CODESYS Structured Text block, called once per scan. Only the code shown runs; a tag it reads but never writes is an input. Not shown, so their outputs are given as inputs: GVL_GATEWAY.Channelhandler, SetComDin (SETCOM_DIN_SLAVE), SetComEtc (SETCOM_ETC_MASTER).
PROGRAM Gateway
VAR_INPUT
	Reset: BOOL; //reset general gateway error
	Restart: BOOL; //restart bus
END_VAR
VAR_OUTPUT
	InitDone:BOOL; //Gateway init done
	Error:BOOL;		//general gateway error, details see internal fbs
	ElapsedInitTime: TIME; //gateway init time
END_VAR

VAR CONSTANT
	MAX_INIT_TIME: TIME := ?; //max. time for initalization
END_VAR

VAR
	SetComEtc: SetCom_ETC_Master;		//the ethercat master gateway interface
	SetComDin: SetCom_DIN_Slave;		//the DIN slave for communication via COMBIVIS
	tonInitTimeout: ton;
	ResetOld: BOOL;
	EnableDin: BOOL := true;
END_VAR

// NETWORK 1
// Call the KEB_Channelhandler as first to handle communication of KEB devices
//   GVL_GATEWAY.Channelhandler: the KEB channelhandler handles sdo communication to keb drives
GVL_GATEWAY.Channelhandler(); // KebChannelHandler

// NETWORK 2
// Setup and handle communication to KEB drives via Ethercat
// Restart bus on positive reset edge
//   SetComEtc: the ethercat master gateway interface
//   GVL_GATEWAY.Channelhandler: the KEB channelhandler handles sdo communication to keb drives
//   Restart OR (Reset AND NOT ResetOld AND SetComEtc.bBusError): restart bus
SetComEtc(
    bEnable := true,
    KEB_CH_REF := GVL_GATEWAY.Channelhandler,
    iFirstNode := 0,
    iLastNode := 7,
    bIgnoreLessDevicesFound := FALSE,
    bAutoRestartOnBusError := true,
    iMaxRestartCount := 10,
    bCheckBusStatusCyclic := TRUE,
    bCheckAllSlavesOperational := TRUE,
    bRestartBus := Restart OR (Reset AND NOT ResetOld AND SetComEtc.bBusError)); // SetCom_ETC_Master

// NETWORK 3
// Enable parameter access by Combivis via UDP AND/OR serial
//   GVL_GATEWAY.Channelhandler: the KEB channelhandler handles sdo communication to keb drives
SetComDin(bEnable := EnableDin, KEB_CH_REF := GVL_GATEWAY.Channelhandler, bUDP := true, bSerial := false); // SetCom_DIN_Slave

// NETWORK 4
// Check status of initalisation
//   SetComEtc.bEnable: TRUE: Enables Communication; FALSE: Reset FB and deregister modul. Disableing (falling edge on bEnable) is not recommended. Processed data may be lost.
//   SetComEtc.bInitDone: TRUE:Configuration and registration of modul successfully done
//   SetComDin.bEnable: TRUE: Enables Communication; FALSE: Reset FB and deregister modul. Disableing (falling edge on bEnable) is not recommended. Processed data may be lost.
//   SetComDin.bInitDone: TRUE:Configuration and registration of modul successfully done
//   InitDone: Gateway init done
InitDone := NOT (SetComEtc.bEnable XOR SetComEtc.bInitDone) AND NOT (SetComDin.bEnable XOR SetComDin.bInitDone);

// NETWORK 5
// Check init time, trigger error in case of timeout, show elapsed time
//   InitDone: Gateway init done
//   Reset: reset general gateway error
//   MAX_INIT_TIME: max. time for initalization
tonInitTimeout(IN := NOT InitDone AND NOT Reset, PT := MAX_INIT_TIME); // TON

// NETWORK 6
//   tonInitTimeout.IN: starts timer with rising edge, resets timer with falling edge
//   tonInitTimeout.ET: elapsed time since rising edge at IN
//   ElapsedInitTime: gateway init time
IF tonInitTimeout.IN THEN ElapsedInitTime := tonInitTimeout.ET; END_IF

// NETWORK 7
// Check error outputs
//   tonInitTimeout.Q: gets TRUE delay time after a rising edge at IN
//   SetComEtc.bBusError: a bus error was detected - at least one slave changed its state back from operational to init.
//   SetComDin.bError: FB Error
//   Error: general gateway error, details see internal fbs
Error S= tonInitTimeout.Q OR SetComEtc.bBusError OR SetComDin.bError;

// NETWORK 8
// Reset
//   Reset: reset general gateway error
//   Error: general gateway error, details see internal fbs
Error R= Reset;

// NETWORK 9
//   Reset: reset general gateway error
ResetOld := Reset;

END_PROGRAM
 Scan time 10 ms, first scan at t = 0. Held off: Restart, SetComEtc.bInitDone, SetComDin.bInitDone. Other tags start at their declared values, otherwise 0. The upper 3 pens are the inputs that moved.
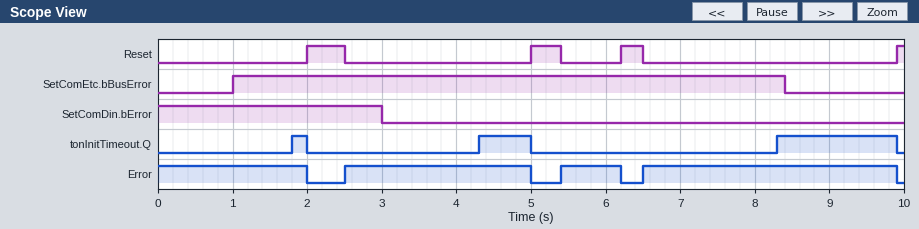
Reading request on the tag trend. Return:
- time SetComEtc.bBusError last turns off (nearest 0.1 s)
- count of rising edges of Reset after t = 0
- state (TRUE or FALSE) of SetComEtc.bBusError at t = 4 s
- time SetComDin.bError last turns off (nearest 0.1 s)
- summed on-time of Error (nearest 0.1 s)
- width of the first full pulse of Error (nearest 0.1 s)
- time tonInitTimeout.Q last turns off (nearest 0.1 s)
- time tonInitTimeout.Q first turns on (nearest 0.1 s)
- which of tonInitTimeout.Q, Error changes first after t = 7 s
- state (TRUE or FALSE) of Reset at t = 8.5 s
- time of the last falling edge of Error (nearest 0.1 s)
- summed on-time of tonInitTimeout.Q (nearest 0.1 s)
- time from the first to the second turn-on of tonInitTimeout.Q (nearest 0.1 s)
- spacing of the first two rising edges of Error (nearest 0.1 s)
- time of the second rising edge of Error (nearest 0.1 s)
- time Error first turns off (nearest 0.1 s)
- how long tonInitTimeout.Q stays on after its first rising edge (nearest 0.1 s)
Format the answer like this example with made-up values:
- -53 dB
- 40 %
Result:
- 8.4 s
- 4
- TRUE
- 3.0 s
- 8.7 s
- 2.5 s
- 9.9 s
- 1.8 s
- tonInitTimeout.Q
- FALSE
- 9.9 s
- 2.5 s
- 2.5 s
- 2.9 s
- 5.4 s
- 2.0 s
- 0.2 s
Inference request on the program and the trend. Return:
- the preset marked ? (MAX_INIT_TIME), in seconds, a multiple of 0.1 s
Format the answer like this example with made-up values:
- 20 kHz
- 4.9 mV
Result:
- 1.8 s
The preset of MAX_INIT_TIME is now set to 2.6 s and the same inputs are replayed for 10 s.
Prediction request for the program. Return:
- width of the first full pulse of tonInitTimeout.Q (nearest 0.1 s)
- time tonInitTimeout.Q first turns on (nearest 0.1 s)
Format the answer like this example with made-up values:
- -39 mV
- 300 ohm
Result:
- 0.8 s
- 9.1 s
